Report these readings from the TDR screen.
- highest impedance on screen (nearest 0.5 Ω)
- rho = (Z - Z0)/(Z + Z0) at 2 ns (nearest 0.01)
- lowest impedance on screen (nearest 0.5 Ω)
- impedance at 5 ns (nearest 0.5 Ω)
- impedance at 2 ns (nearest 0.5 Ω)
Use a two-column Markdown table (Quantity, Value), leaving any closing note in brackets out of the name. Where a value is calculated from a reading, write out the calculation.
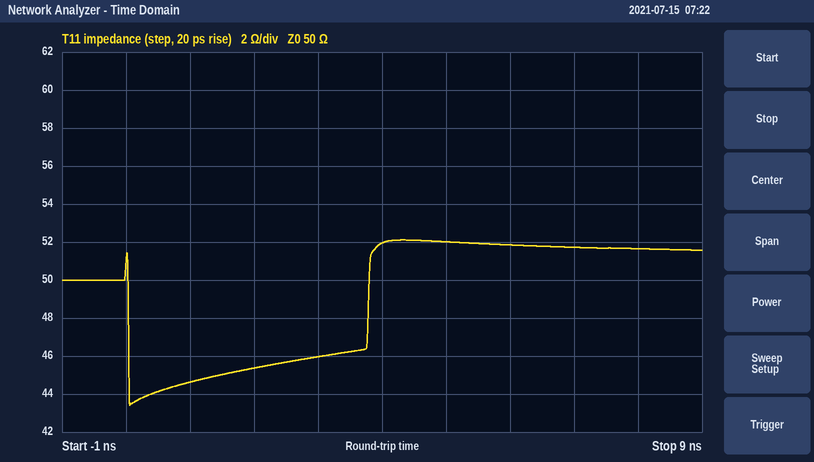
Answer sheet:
| Quantity | Value |
|---|---|
| highest impedance on screen | 52.0 Ω |
| rho = (Z - Z0)/(Z + Z0) at 2 ns | (45.5 − 50)/(45.5 + 50) ≈ -0.05 |
| lowest impedance on screen | 43.5 Ω |
| impedance at 5 ns | 52.0 Ω |
| impedance at 2 ns | 45.5 Ω |
